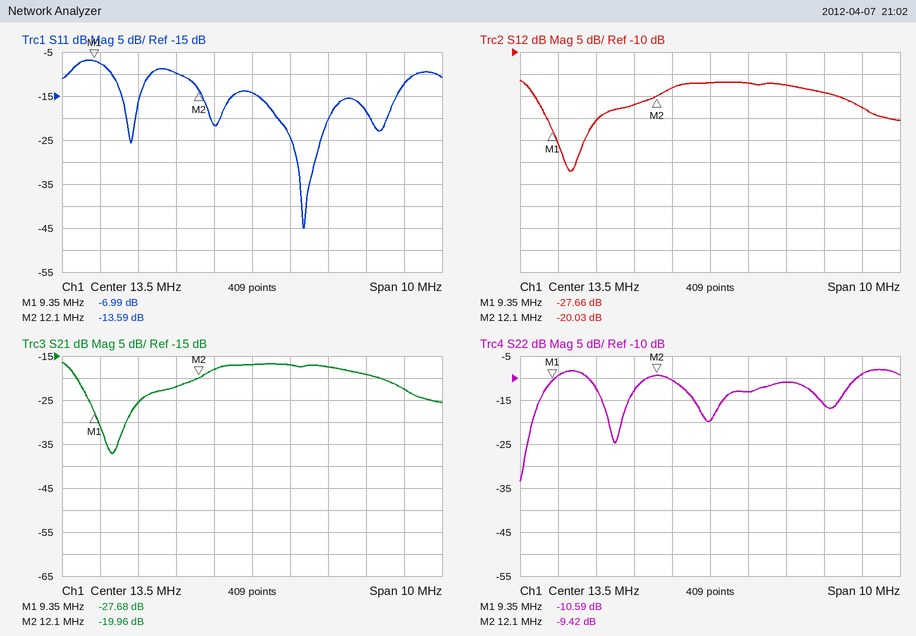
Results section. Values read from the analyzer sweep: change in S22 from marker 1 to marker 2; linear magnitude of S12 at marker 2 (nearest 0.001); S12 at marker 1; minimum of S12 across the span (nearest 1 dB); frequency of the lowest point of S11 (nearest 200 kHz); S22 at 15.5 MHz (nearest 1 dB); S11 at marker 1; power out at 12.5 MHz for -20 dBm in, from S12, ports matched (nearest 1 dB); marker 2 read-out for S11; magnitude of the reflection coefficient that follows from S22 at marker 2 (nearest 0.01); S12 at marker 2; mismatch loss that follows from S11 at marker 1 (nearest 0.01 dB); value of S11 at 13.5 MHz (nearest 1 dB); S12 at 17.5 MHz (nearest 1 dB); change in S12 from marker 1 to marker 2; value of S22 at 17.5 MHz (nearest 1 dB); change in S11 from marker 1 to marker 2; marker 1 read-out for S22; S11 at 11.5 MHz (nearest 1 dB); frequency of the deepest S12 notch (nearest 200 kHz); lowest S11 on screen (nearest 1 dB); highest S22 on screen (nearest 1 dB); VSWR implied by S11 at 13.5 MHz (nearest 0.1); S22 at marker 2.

1.17 dB
0.100
-27.66 dB
-37 dB
14.8 MHz
-11 dB
-6.99 dB
-38 dBm
-13.59 dB
0.34
-20.03 dB
0.97 dB
-14 dB
-23 dB
7.63 dB
-9 dB
-6.60 dB
-10.59 dB
-10 dB
9.8 MHz
-45 dB
-8 dB
1.5
-9.42 dB
